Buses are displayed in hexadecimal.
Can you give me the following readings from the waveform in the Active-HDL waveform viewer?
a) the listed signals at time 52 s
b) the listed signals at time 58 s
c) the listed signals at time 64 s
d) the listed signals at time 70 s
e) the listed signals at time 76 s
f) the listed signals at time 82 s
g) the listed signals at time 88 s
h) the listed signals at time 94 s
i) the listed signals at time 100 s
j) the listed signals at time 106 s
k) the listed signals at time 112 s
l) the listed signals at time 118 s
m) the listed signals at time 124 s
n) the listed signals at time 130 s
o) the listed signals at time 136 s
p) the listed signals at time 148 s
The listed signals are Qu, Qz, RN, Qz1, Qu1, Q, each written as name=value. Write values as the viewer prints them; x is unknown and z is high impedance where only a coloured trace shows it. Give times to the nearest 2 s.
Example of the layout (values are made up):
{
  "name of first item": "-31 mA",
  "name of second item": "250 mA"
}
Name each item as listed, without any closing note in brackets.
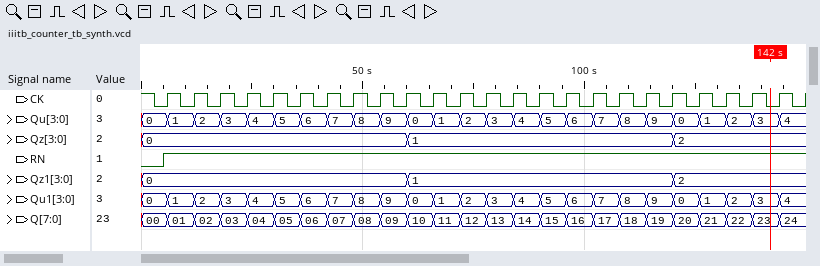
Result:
{
  "the listed signals at time 52 s": "Qu=8, Qz=0, RN=1, Qz1=0, Qu1=8, Q=08",
  "the listed signals at time 58 s": "Qu=9, Qz=0, RN=1, Qz1=0, Qu1=9, Q=09",
  "the listed signals at time 64 s": "Qu=0, Qz=1, RN=1, Qz1=1, Qu1=0, Q=10",
  "the listed signals at time 70 s": "Qu=1, Qz=1, RN=1, Qz1=1, Qu1=1, Q=11",
  "the listed signals at time 76 s": "Qu=2, Qz=1, RN=1, Qz1=1, Qu1=2, Q=12",
  "the listed signals at time 82 s": "Qu=3, Qz=1, RN=1, Qz1=1, Qu1=3, Q=13",
  "the listed signals at time 88 s": "Qu=4, Qz=1, RN=1, Qz1=1, Qu1=4, Q=14",
  "the listed signals at time 94 s": "Qu=5, Qz=1, RN=1, Qz1=1, Qu1=5, Q=15",
  "the listed signals at time 100 s": "Qu=6, Qz=1, RN=1, Qz1=1, Qu1=6, Q=16",
  "the listed signals at time 106 s": "Qu=7, Qz=1, RN=1, Qz1=1, Qu1=7, Q=17",
  "the listed signals at time 112 s": "Qu=8, Qz=1, RN=1, Qz1=1, Qu1=8, Q=18",
  "the listed signals at time 118 s": "Qu=9, Qz=1, RN=1, Qz1=1, Qu1=9, Q=19",
  "the listed signals at time 124 s": "Qu=0, Qz=2, RN=1, Qz1=2, Qu1=0, Q=20",
  "the listed signals at time 130 s": "Qu=1, Qz=2, RN=1, Qz1=2, Qu1=1, Q=21",
  "the listed signals at time 136 s": "Qu=2, Qz=2, RN=1, Qz1=2, Qu1=2, Q=22",
  "the listed signals at time 148 s": "Qu=4, Qz=2, RN=1, Qz1=2, Qu1=4, Q=24"
}
